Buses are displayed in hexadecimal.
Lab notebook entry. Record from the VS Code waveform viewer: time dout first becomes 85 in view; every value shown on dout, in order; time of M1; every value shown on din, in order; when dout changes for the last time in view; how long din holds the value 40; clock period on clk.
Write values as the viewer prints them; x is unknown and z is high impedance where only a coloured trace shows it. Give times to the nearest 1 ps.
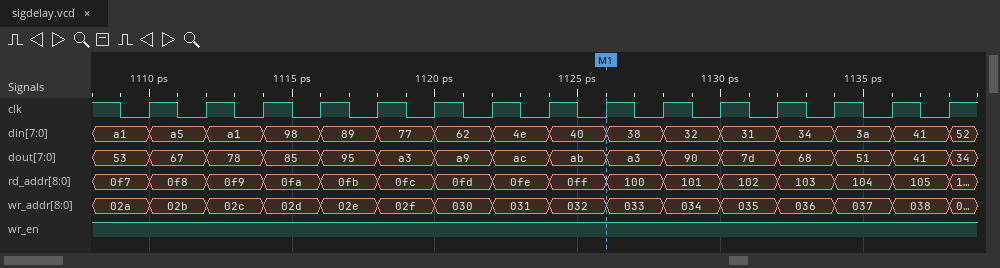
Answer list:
1114 ps
53, 67, 78, 85, 95, a3, a9, ac, ab, a3, 90, 7d, 68, 51, 41, 34
1126 ps
a1, a5, a1, 98, 89, 77, 62, 4e, 40, 38, 32, 31, 34, 3a, 41, 52
1138 ps
2 ps
2 ps
